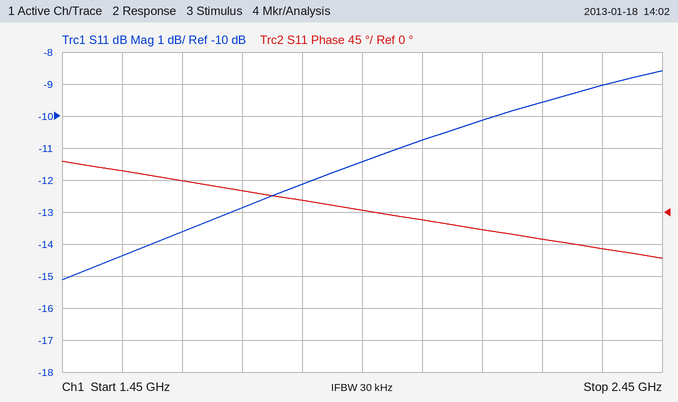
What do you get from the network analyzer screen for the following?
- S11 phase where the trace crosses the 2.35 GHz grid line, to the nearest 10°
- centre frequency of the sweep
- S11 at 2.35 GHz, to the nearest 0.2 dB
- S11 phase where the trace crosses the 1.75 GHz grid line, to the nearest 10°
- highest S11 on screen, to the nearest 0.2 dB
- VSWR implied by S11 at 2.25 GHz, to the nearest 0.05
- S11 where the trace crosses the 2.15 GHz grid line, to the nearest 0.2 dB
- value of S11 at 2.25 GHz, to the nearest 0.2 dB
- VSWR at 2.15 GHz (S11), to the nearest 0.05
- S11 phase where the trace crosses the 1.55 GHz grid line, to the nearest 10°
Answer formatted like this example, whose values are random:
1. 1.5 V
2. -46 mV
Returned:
1. -50°
2. 1.95 GHz
3. -9.0 dB
4. 30°
5. -8.6 dB
6. 2.00
7. -10.2 dB
8. -9.6 dB
9. 1.90
10. 60°
